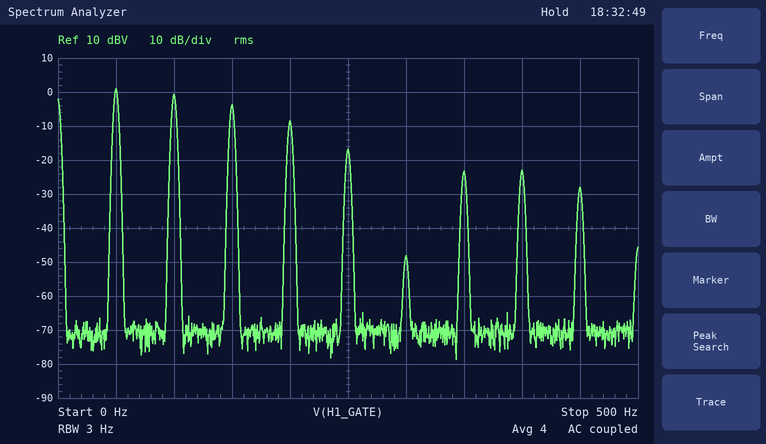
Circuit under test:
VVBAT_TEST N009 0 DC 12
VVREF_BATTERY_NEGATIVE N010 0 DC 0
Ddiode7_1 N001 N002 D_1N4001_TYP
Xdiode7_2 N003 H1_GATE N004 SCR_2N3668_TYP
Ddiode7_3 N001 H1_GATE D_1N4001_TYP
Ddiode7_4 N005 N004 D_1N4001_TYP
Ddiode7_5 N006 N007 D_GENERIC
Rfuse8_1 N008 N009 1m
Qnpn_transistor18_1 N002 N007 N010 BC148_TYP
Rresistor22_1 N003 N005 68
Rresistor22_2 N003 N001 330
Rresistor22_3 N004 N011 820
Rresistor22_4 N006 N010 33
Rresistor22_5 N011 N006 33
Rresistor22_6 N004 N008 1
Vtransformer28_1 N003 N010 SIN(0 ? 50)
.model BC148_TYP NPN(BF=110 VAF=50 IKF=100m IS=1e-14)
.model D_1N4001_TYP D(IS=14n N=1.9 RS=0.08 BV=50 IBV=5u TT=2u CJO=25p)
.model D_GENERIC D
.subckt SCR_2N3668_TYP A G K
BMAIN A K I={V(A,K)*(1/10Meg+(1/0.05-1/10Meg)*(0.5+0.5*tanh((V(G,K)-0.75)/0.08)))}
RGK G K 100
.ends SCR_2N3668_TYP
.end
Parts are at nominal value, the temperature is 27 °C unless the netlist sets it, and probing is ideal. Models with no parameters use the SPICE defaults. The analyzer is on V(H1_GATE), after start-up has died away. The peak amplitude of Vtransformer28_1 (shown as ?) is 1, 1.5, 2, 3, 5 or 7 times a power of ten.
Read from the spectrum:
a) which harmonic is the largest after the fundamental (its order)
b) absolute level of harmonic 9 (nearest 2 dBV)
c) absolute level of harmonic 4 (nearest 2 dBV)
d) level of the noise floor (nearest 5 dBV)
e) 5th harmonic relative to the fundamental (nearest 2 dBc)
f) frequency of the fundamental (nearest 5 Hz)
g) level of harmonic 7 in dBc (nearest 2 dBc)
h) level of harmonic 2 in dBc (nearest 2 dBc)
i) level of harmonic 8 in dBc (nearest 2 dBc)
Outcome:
2
-28 dBV
-8 dBV
-70 dBV
-18 dBc
50 Hz
-24 dBc
-2 dBc
-24 dBc
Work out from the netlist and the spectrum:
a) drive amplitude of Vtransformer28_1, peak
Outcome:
20 V
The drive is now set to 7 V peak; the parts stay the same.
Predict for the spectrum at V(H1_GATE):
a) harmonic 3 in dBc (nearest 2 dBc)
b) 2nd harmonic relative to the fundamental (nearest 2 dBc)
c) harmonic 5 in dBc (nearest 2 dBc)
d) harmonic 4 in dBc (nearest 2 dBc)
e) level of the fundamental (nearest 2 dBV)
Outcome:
-34 dBc
-20 dBc
-58 dBc
-46 dBc
-116 dBV
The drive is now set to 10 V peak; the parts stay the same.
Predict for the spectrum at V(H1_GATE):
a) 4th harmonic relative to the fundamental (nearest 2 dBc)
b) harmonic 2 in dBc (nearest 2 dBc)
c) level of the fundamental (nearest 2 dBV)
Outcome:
-34 dBc
-16 dBc
-112 dBV
